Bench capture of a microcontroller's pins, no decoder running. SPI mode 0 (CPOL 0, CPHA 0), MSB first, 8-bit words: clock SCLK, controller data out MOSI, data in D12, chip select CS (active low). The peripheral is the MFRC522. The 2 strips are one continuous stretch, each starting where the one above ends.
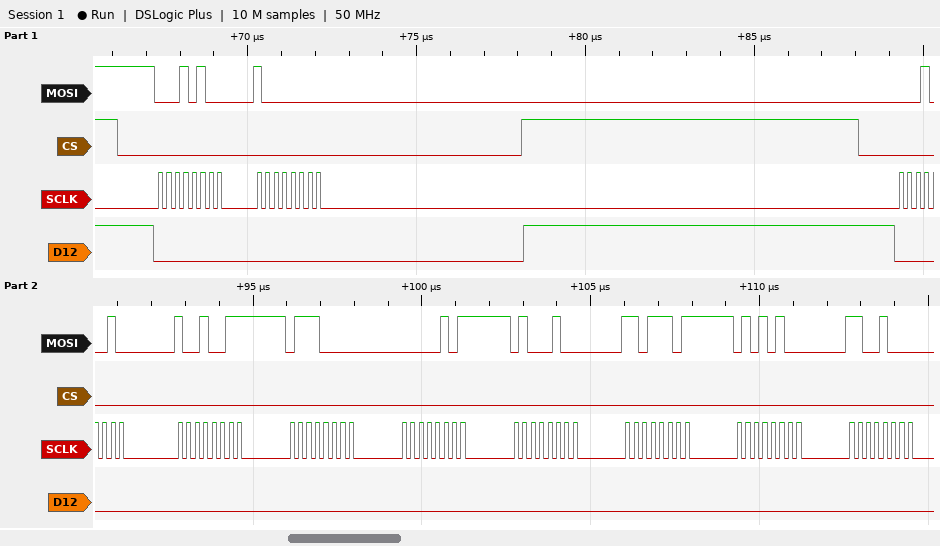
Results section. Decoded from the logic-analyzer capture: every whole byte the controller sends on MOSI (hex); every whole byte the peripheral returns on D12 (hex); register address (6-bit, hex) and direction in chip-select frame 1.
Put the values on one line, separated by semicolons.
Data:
14 80 12 93 70 05 44 DD 54 C8; 00 00 00 00 00 00 00 00 00 00; 0x0A write
